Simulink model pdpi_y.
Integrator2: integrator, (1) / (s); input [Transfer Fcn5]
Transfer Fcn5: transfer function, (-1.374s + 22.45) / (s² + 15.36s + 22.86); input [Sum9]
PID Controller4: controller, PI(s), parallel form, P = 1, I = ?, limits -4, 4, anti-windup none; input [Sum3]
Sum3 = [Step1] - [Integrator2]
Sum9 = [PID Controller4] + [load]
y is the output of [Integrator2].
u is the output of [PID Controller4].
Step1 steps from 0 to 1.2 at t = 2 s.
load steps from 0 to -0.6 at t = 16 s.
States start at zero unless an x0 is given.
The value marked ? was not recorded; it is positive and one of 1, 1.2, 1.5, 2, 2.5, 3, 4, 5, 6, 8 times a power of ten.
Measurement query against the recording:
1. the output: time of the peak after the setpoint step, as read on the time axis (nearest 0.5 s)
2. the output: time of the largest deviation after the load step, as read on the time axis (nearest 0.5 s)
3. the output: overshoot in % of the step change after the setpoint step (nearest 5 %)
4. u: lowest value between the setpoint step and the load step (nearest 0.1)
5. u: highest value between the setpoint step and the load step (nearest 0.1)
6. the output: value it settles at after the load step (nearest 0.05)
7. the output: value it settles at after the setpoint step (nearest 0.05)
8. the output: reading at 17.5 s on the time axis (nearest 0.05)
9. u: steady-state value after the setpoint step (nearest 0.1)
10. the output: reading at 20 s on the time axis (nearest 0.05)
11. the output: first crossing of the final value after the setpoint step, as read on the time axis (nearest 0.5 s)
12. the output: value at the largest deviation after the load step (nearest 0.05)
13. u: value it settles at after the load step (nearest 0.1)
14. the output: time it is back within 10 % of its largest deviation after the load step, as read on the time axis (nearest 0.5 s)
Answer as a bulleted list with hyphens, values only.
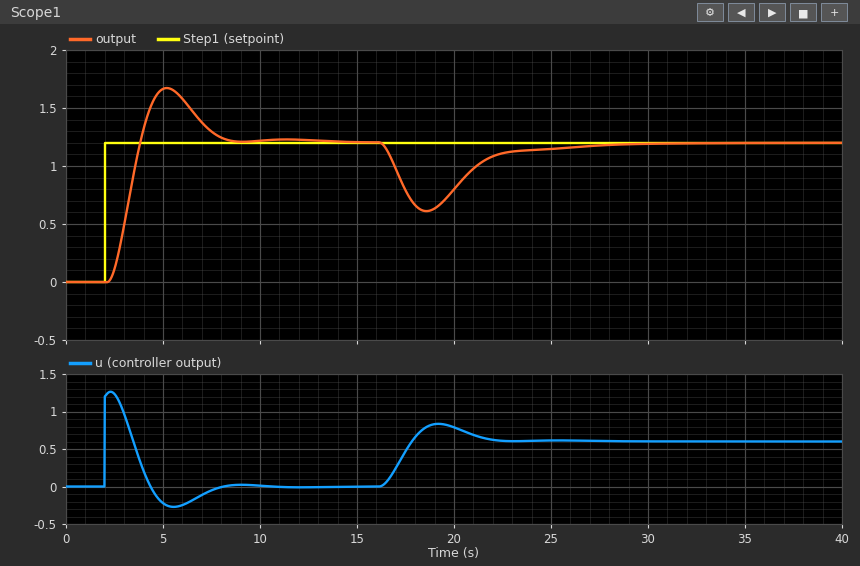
- 5.0 s
- 18.5 s
- 40 %
- -0.3
- 1.3
- 1.20
- 1.20
- 0.80
- 0.0
- 0.80
- 4.0 s
- 0.60
- 0.6
- 24.5 s
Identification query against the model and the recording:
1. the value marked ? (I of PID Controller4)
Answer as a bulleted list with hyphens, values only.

- 0.25
